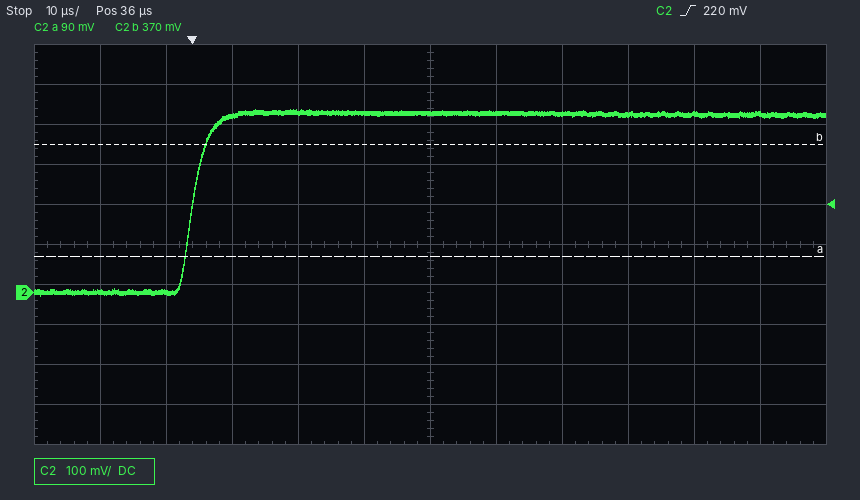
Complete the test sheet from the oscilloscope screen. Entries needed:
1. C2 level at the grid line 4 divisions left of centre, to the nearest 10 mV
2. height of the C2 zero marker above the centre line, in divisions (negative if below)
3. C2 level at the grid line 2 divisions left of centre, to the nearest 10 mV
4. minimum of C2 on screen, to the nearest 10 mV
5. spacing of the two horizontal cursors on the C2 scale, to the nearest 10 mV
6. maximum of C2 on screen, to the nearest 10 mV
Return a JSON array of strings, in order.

["0 mV", "-1.2 div", "450 mV", "-10 mV", "280 mV", "460 mV"]
